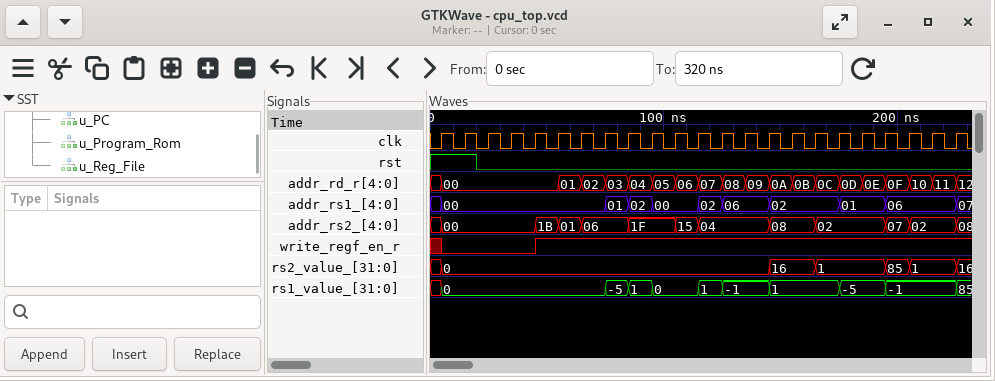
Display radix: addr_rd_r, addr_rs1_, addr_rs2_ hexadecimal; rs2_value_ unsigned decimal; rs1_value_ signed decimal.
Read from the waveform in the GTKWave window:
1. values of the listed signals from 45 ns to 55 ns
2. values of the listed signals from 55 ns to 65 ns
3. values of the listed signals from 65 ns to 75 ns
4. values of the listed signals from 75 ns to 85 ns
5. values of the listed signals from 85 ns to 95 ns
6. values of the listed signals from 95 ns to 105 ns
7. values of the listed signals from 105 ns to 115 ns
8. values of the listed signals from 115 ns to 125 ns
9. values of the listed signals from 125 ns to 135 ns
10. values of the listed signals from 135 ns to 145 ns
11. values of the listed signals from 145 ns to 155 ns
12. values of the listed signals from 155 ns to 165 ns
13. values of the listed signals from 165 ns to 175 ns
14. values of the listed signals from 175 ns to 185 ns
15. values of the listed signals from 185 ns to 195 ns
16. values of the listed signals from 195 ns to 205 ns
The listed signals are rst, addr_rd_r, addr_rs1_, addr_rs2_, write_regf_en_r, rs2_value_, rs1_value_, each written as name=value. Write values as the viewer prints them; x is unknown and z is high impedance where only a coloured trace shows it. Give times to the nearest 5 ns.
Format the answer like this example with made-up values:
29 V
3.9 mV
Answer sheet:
rst=0, addr_rd_r=00, addr_rs1_=00, addr_rs2_=1B, write_regf_en_r=1, rs2_value_=0, rs1_value_=0
rst=0, addr_rd_r=01, addr_rs1_=00, addr_rs2_=01, write_regf_en_r=1, rs2_value_=0, rs1_value_=0
rst=0, addr_rd_r=02, addr_rs1_=00, addr_rs2_=06, write_regf_en_r=1, rs2_value_=0, rs1_value_=0
rst=0, addr_rd_r=03, addr_rs1_=01, addr_rs2_=06, write_regf_en_r=1, rs2_value_=0, rs1_value_=-5
rst=0, addr_rd_r=04, addr_rs1_=02, addr_rs2_=1F, write_regf_en_r=1, rs2_value_=0, rs1_value_=1
rst=0, addr_rd_r=05, addr_rs1_=00, addr_rs2_=1F, write_regf_en_r=1, rs2_value_=0, rs1_value_=0
rst=0, addr_rd_r=06, addr_rs1_=00, addr_rs2_=15, write_regf_en_r=1, rs2_value_=0, rs1_value_=0
rst=0, addr_rd_r=07, addr_rs1_=02, addr_rs2_=04, write_regf_en_r=1, rs2_value_=0, rs1_value_=1
rst=0, addr_rd_r=08, addr_rs1_=06, addr_rs2_=04, write_regf_en_r=1, rs2_value_=0, rs1_value_=-1
rst=0, addr_rd_r=09, addr_rs1_=06, addr_rs2_=04, write_regf_en_r=1, rs2_value_=0, rs1_value_=-1
rst=0, addr_rd_r=0A, addr_rs1_=02, addr_rs2_=08, write_regf_en_r=1, rs2_value_=16, rs1_value_=1
rst=0, addr_rd_r=0B, addr_rs1_=02, addr_rs2_=08, write_regf_en_r=1, rs2_value_=16, rs1_value_=1
rst=0, addr_rd_r=0C, addr_rs1_=02, addr_rs2_=02, write_regf_en_r=1, rs2_value_=1, rs1_value_=1
rst=0, addr_rd_r=0D, addr_rs1_=01, addr_rs2_=02, write_regf_en_r=1, rs2_value_=1, rs1_value_=-5
rst=0, addr_rd_r=0E, addr_rs1_=01, addr_rs2_=02, write_regf_en_r=1, rs2_value_=1, rs1_value_=-5
rst=0, addr_rd_r=0F, addr_rs1_=06, addr_rs2_=07, write_regf_en_r=1, rs2_value_=85, rs1_value_=-1
